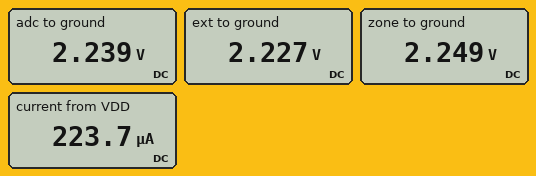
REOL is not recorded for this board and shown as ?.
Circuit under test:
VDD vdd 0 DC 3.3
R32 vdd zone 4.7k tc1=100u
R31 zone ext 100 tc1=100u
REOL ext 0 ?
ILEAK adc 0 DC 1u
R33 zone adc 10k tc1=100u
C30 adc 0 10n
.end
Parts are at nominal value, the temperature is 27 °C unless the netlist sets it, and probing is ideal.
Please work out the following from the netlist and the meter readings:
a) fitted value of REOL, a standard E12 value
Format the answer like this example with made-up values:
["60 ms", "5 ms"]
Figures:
["10 kΩ"]
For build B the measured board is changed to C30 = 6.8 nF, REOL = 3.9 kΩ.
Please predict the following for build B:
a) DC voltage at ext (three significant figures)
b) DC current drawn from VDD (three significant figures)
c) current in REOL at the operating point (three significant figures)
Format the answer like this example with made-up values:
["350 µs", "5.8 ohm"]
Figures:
["1.48 V", "380 µA", "379 µA"]
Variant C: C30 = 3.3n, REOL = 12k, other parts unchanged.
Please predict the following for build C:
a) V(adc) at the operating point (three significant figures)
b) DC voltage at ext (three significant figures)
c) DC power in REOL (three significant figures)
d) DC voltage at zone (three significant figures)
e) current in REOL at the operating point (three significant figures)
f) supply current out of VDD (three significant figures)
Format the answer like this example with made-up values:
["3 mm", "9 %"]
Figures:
["2.36 V", "2.35 V", "462 µW", "2.37 V", "196 µA", "197 µA"]
